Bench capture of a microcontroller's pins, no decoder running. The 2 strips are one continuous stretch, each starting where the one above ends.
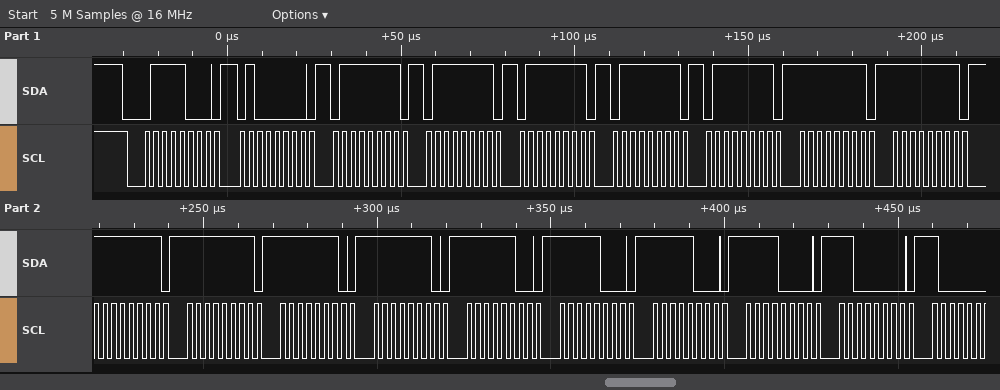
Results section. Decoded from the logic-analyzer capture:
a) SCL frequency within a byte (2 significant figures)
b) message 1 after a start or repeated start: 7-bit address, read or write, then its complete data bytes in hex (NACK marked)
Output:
400 kHz
0x3C write: 40 7F 7F 7F 7F 7F FF FF FF FF FE FE FC F8 F8 F0 C0
